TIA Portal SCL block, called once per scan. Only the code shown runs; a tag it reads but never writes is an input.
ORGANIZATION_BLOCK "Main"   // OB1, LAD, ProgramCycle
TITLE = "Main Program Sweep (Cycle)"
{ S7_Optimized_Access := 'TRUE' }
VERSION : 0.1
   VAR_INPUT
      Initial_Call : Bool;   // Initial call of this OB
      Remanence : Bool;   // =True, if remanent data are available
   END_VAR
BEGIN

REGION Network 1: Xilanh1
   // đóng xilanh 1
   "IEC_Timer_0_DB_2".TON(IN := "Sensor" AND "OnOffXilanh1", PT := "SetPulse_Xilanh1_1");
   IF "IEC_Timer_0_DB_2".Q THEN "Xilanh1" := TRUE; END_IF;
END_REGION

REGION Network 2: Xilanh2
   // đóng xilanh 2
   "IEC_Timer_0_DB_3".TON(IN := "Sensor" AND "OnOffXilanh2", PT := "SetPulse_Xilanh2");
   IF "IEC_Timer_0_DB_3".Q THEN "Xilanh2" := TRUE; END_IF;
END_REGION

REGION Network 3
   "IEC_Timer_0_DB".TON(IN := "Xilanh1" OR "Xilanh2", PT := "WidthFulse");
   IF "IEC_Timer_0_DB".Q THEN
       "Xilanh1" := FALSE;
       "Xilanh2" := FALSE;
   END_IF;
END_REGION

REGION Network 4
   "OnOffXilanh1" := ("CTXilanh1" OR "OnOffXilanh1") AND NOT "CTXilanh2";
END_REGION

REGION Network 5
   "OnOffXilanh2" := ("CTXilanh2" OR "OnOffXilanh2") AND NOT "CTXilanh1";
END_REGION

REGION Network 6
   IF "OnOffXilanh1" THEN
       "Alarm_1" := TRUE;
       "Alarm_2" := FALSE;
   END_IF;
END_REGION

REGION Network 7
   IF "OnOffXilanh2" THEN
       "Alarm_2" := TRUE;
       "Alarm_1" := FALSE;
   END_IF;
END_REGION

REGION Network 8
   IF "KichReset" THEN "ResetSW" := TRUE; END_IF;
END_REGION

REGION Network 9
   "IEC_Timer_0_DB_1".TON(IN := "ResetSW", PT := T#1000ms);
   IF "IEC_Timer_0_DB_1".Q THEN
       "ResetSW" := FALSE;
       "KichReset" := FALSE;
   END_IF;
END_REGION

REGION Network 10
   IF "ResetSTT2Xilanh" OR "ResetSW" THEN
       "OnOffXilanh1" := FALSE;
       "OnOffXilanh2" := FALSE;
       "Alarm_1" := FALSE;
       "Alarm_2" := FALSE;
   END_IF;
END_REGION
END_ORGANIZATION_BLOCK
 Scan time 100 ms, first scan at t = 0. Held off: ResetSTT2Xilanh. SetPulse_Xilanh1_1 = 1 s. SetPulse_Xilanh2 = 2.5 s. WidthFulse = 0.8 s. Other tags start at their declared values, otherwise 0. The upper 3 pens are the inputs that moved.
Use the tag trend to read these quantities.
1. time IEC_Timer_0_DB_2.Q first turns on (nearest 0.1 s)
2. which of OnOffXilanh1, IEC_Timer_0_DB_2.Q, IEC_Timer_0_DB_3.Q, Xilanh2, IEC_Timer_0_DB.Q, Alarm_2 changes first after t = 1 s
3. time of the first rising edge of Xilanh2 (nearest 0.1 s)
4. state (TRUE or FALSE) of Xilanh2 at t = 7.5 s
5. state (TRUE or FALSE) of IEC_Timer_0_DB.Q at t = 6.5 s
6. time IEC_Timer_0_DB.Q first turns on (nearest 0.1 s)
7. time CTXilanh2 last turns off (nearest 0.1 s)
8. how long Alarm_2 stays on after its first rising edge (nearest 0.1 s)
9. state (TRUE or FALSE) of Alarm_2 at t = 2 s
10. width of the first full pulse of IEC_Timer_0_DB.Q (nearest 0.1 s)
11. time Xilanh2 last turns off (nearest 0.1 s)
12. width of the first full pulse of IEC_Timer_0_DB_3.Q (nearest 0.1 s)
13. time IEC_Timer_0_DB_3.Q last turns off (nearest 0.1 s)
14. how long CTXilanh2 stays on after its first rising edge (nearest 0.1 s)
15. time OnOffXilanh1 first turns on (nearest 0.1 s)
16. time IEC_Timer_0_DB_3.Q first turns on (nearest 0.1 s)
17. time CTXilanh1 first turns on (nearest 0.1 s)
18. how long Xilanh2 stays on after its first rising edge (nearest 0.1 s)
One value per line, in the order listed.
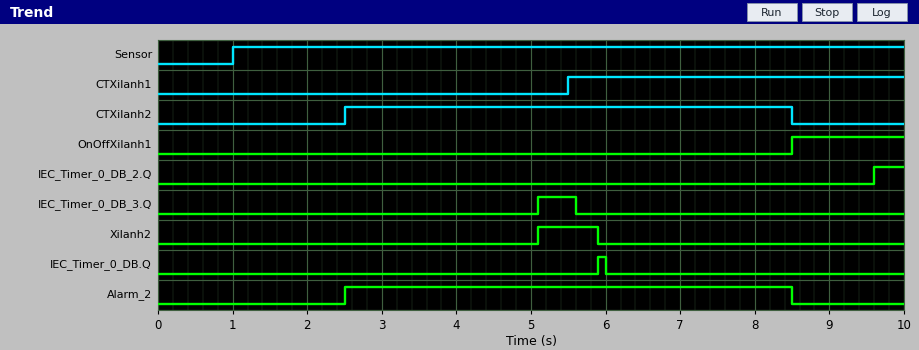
9.6 s
Alarm_2
5.1 s
FALSE
FALSE
5.9 s
8.5 s
6.0 s
FALSE
0.1 s
5.9 s
0.5 s
5.6 s
6.0 s
8.5 s
5.1 s
5.5 s
0.8 s
